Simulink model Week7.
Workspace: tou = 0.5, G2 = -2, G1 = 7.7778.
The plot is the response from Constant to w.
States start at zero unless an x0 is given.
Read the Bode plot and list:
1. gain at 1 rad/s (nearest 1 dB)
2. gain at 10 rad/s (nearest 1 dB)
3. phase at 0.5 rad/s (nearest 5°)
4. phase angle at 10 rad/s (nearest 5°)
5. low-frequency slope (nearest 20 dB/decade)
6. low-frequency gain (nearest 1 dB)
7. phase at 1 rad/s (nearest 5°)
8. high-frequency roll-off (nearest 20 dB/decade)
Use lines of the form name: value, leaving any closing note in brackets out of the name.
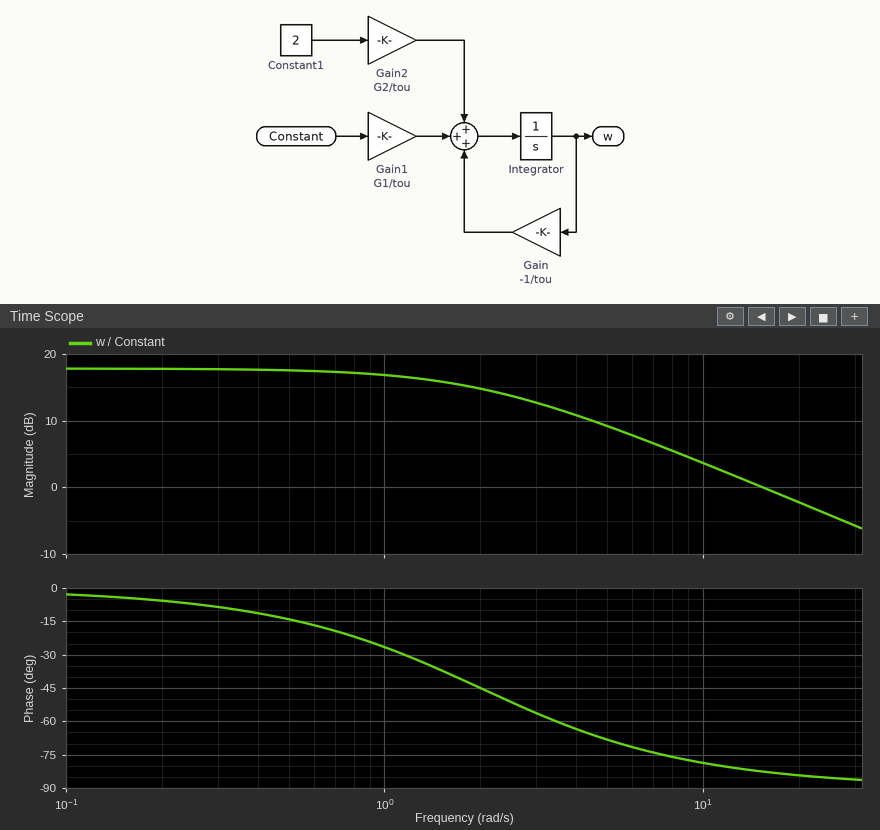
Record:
gain at 1 rad/s: 17 dB
gain at 10 rad/s: 4 dB
phase at 0.5 rad/s: -15°
phase angle at 10 rad/s: -80°
low-frequency slope: 0 dB/decade
low-frequency gain: 18 dB
phase at 1 rad/s: -25°
high-frequency roll-off: -20 dB/decade
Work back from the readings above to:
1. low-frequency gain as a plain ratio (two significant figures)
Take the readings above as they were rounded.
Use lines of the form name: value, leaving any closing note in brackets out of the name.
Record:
low-frequency gain as a plain ratio: 7.9
